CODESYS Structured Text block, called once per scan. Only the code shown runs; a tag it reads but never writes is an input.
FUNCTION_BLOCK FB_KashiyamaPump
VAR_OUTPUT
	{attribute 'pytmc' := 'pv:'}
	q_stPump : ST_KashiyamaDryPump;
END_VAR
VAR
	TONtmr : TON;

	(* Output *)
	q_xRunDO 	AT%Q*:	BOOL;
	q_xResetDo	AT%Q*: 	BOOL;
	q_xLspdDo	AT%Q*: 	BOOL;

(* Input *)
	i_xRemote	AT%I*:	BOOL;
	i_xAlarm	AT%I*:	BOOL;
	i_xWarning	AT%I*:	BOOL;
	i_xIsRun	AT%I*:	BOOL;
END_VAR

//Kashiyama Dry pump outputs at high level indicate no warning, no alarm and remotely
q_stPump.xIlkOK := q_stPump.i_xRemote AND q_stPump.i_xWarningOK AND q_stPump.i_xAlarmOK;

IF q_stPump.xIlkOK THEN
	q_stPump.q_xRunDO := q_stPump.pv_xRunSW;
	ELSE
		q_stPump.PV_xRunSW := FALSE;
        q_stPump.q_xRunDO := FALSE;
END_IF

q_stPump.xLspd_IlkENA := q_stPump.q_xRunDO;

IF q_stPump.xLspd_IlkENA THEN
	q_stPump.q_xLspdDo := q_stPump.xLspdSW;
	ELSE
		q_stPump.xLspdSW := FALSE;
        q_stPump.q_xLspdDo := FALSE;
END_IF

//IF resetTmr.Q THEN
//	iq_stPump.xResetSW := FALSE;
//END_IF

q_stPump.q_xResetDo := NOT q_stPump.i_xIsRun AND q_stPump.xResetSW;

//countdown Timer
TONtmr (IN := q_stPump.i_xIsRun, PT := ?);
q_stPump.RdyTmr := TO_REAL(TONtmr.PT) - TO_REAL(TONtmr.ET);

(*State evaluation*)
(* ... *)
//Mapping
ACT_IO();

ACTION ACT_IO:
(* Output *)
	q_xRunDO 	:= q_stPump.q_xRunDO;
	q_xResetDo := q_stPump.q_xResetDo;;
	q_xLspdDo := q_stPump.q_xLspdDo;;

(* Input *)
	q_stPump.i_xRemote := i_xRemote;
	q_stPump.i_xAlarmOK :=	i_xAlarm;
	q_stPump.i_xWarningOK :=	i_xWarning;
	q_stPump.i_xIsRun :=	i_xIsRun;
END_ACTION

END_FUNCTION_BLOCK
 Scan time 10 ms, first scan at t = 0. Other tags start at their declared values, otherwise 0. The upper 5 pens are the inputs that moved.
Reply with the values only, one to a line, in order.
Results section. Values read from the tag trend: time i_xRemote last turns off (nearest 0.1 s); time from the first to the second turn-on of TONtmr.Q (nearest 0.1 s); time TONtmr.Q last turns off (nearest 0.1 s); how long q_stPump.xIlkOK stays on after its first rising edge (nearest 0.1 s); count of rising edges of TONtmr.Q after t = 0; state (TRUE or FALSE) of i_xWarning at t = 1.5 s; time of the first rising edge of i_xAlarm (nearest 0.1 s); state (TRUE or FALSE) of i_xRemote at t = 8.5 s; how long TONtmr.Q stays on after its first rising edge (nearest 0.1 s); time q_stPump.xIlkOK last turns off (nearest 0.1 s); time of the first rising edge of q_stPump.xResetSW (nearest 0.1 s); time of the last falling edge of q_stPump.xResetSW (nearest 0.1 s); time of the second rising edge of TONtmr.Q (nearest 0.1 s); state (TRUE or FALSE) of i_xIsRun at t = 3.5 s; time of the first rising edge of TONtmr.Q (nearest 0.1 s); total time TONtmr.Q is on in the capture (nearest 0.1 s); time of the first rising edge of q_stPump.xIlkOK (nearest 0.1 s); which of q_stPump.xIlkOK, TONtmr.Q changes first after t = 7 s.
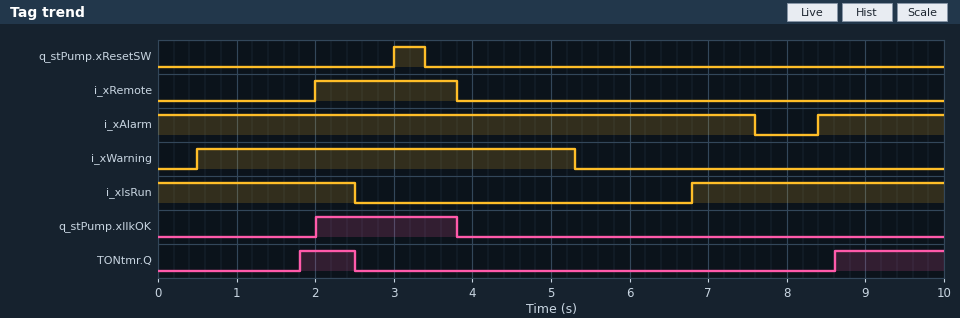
3.8 s
6.8 s
2.5 s
1.8 s
2
TRUE
8.4 s
FALSE
0.7 s
3.8 s
3.0 s
3.4 s
8.6 s
FALSE
1.8 s
2.1 s
2.0 s
TONtmr.Q
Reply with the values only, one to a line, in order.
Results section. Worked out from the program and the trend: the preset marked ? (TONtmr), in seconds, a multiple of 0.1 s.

1.8 s
